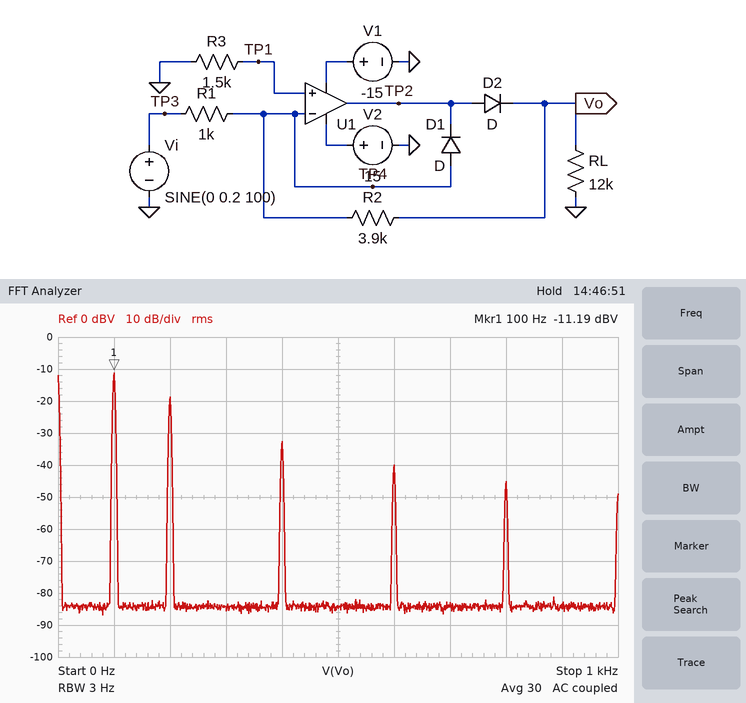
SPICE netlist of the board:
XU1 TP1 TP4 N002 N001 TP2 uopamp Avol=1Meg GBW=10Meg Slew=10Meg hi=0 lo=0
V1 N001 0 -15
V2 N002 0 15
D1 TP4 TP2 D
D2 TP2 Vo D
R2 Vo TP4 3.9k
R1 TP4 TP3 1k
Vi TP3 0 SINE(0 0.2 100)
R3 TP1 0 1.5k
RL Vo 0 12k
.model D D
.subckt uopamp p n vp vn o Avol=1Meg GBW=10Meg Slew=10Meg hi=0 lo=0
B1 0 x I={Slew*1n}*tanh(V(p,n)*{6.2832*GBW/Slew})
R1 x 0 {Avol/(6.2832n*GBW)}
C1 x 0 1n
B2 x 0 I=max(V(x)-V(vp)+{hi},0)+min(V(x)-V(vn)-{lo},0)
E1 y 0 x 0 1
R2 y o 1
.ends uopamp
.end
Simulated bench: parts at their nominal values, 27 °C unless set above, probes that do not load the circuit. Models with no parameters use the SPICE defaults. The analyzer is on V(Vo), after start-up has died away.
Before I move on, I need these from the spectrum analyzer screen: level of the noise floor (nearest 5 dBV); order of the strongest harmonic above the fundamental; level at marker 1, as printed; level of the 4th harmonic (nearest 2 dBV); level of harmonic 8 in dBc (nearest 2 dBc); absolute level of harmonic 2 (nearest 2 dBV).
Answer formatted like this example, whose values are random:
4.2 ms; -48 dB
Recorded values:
-85 dBV; 2; -11.19 dBV; -32 dBV; -34 dBc; -18 dBV
